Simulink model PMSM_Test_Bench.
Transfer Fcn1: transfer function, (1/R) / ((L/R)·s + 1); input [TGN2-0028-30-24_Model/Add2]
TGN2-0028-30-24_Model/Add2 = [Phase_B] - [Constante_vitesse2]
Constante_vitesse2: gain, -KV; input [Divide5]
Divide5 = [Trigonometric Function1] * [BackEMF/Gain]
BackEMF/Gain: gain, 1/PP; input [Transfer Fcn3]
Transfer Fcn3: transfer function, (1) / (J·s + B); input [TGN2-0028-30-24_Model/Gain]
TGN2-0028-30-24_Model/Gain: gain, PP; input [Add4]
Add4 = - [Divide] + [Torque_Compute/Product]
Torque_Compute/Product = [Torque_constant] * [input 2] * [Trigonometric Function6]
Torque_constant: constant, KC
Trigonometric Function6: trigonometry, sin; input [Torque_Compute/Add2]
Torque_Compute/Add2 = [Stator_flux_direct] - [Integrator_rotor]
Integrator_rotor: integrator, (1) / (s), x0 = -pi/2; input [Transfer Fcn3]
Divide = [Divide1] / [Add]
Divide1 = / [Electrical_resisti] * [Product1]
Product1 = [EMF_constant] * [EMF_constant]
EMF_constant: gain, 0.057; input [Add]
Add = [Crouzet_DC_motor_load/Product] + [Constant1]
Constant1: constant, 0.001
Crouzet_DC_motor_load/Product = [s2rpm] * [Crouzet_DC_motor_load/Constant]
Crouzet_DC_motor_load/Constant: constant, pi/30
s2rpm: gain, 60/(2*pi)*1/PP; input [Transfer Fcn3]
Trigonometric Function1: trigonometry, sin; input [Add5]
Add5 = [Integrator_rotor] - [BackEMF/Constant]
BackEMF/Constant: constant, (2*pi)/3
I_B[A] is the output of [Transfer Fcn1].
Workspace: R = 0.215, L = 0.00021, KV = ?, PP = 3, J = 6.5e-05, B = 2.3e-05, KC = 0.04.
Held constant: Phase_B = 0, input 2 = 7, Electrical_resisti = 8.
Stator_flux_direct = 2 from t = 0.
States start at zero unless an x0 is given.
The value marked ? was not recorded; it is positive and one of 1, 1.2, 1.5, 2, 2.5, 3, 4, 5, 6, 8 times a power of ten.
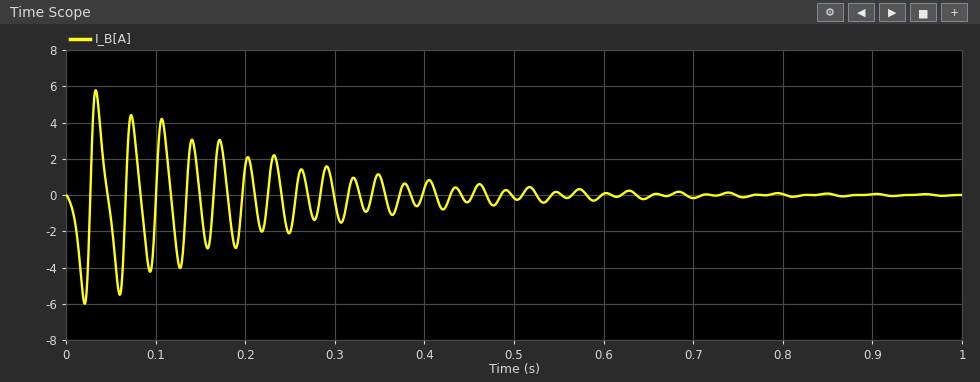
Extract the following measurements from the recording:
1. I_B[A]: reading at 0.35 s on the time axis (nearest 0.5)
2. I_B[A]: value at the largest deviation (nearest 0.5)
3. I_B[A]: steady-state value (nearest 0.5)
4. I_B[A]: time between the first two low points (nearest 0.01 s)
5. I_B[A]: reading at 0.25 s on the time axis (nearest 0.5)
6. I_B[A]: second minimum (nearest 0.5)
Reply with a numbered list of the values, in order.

1. 1.0
2. -6.0
3. 0.0
4. 0.04 s
5. -2.0
6. -5.5
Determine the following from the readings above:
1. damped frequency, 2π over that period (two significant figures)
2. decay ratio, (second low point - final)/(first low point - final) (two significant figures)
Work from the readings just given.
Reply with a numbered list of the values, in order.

1. 160 rad/s
2. 0.92
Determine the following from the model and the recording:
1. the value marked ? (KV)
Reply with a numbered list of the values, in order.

1. 0.025
